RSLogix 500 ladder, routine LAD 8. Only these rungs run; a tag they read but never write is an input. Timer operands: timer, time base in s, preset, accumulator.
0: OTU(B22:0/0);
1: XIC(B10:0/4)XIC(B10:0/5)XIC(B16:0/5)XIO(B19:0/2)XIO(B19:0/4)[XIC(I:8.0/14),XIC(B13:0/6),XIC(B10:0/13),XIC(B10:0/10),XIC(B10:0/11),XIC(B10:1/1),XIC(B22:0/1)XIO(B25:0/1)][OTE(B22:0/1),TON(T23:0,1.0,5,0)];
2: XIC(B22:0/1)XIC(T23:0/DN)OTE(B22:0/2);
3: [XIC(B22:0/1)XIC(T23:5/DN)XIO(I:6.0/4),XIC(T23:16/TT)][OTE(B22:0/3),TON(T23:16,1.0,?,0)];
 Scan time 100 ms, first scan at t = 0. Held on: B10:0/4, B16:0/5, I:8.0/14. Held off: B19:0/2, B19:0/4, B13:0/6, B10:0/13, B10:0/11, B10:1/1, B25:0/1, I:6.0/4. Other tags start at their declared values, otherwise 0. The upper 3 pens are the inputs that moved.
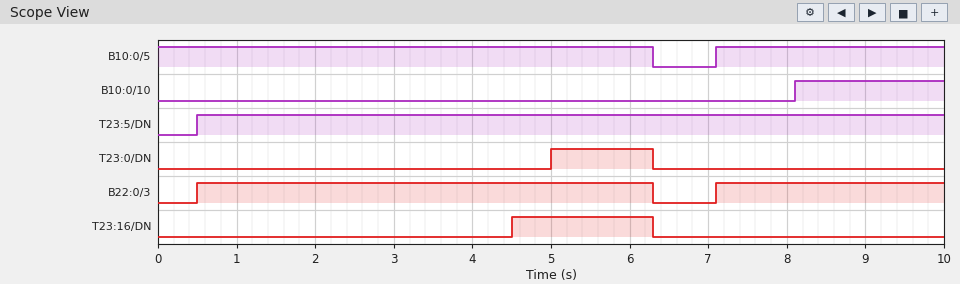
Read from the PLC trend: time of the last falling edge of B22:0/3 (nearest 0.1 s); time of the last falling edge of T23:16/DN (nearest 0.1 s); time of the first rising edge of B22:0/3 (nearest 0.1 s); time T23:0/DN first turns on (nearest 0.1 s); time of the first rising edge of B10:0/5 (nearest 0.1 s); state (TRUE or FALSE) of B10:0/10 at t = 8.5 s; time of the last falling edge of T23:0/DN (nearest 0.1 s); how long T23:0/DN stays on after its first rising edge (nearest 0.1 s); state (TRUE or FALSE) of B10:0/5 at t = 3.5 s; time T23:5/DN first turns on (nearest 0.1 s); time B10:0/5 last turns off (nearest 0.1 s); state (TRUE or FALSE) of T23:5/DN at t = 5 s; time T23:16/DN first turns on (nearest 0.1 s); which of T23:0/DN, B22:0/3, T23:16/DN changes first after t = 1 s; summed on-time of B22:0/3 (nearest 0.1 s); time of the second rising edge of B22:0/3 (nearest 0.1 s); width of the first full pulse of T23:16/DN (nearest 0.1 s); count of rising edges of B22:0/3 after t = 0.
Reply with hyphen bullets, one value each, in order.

- 6.3 s
- 6.3 s
- 0.5 s
- 5.0 s
- 7.1 s
- TRUE
- 6.3 s
- 1.3 s
- TRUE
- 0.5 s
- 6.3 s
- TRUE
- 4.5 s
- T23:16/DN
- 8.7 s
- 7.1 s
- 1.8 s
- 2
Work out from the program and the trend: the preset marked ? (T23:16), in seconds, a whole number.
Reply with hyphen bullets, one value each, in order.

- 4 s
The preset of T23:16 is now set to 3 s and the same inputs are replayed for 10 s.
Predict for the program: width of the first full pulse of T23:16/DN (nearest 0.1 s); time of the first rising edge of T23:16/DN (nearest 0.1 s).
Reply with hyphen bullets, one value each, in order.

- 2.8 s
- 3.5 s
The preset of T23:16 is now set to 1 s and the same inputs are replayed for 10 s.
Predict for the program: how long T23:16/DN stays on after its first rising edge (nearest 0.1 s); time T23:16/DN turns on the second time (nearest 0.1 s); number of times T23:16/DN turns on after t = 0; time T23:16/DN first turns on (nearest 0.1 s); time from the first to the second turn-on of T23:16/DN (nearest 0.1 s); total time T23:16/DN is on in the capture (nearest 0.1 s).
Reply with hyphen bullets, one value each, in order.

- 4.8 s
- 8.1 s
- 2
- 1.5 s
- 6.6 s
- 6.7 s
